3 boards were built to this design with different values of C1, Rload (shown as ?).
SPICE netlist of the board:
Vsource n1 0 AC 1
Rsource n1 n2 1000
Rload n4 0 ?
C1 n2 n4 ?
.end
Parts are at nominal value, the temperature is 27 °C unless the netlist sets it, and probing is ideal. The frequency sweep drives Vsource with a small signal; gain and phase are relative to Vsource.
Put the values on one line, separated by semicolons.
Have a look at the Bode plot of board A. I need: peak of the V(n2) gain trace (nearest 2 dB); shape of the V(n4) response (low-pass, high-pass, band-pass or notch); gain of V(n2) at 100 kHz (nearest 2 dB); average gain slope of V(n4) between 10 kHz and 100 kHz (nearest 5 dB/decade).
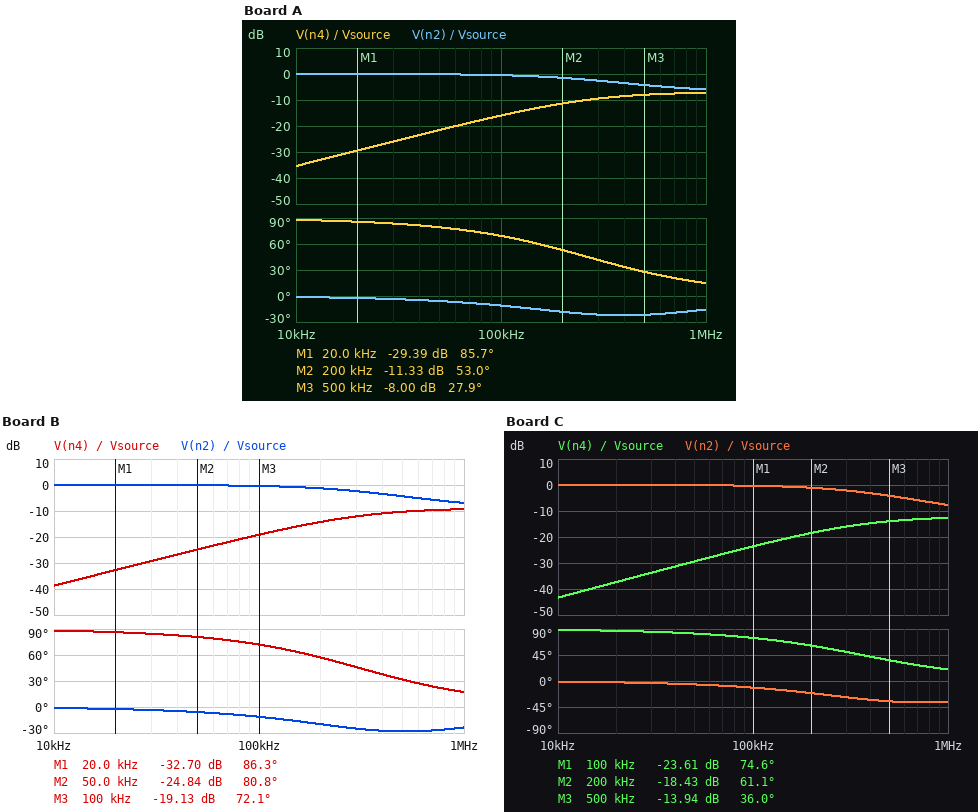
0 dB; high-pass; 0 dB; 20 dB/decade
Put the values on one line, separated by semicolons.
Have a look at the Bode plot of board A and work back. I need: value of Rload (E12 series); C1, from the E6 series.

820 Ω; 330 pF
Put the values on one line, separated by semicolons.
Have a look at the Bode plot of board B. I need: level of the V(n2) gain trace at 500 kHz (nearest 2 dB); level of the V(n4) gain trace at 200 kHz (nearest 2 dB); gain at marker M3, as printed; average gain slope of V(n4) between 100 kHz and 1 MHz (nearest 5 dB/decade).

-4 dB; -14 dB; -19.13 dB; 10 dB/decade
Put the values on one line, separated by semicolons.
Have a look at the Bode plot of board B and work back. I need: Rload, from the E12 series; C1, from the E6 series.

560 Ω; 330 pF
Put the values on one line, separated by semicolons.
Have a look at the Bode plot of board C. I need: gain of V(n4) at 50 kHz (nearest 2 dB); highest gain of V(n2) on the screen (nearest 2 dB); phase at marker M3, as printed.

-30 dB; 0 dB; 36.0 deg
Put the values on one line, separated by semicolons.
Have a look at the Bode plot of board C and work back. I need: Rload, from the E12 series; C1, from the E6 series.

330 Ω; 330 pF
